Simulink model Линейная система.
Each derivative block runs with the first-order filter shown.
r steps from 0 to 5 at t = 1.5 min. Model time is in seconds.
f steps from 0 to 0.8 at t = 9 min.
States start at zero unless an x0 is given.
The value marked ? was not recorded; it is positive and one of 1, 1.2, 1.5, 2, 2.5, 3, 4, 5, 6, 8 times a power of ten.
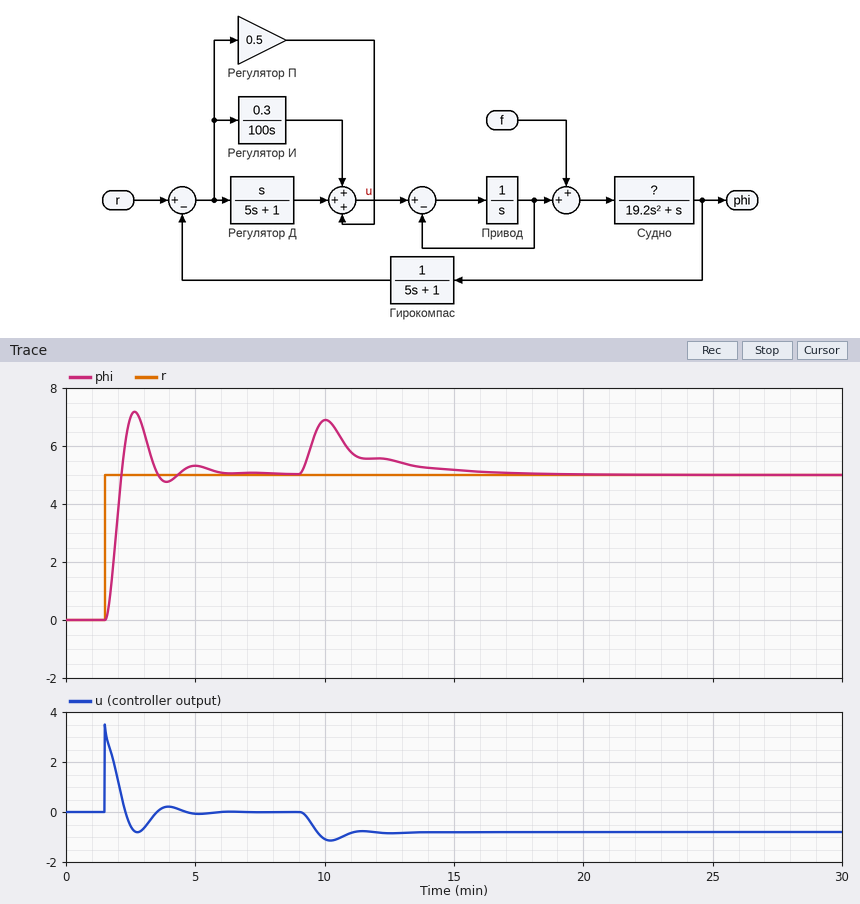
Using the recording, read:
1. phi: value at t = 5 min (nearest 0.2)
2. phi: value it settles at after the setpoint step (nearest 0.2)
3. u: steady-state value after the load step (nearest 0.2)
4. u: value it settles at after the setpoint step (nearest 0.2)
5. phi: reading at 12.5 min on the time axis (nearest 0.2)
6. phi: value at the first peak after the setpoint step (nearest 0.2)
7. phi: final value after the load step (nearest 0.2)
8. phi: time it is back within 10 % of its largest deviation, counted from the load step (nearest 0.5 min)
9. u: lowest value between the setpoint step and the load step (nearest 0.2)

5.4
5.0
-0.8
0.0
5.6
7.2
5.0
6.0 min
-0.8
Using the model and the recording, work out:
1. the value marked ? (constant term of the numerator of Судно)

0.1
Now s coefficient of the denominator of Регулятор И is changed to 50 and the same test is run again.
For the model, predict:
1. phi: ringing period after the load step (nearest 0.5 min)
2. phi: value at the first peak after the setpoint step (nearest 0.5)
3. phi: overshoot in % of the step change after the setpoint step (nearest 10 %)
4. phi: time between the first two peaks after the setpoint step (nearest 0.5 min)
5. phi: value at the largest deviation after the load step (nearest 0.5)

2.5 min
8.0
60 %
2.5 min
7.0
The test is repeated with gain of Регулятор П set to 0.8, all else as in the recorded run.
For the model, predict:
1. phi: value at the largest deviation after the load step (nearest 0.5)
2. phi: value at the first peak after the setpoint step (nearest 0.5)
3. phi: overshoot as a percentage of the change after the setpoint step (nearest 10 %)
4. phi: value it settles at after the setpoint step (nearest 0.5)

6.5
8.0
60 %
5.0
